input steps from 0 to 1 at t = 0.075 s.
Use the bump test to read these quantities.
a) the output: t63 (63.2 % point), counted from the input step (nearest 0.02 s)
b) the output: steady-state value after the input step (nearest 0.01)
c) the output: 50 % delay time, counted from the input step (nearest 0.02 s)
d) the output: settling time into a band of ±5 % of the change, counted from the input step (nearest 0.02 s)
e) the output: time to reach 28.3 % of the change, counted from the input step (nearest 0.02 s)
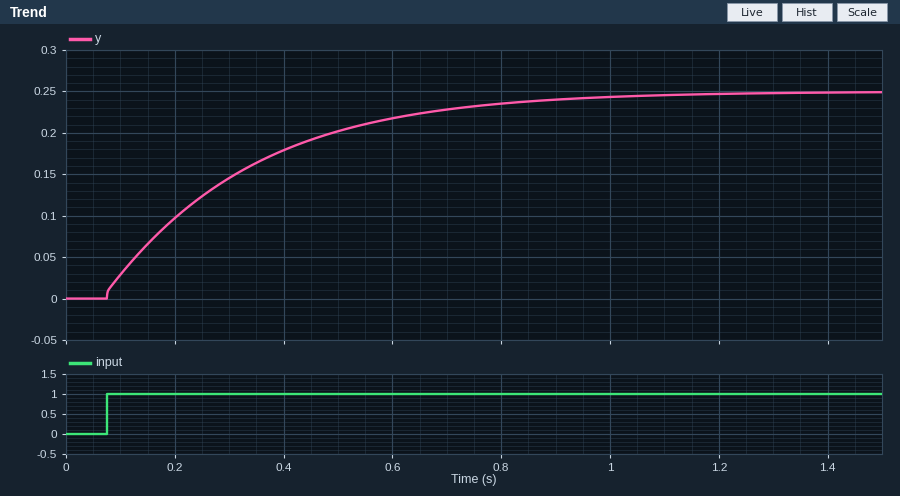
0.26 s
0.25
0.18 s
0.76 s
0.08 s
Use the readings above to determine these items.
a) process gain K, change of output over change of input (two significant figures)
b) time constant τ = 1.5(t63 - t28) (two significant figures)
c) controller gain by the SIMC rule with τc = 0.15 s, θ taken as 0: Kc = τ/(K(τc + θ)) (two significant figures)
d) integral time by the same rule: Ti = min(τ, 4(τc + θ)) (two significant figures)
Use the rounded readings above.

0.25
0.27 s
7.2
0.27 s
